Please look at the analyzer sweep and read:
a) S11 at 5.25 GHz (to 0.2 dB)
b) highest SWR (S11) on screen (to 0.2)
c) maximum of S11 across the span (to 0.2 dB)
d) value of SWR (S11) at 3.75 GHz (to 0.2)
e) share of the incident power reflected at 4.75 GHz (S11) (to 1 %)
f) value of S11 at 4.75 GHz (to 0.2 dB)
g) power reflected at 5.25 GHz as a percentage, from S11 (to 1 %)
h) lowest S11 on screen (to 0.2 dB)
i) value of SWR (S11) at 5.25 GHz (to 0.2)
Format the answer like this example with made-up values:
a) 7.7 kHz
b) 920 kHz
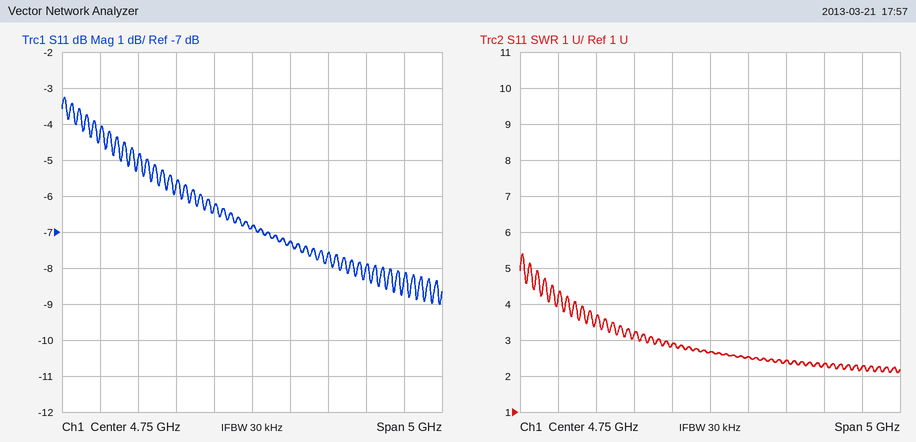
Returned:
a) -7.2 dB
b) 5.4
c) -3.2 dB
d) 3.2
e) 21 %
f) -6.8 dB
g) 19 %
h) -9.0 dB
i) 2.6
